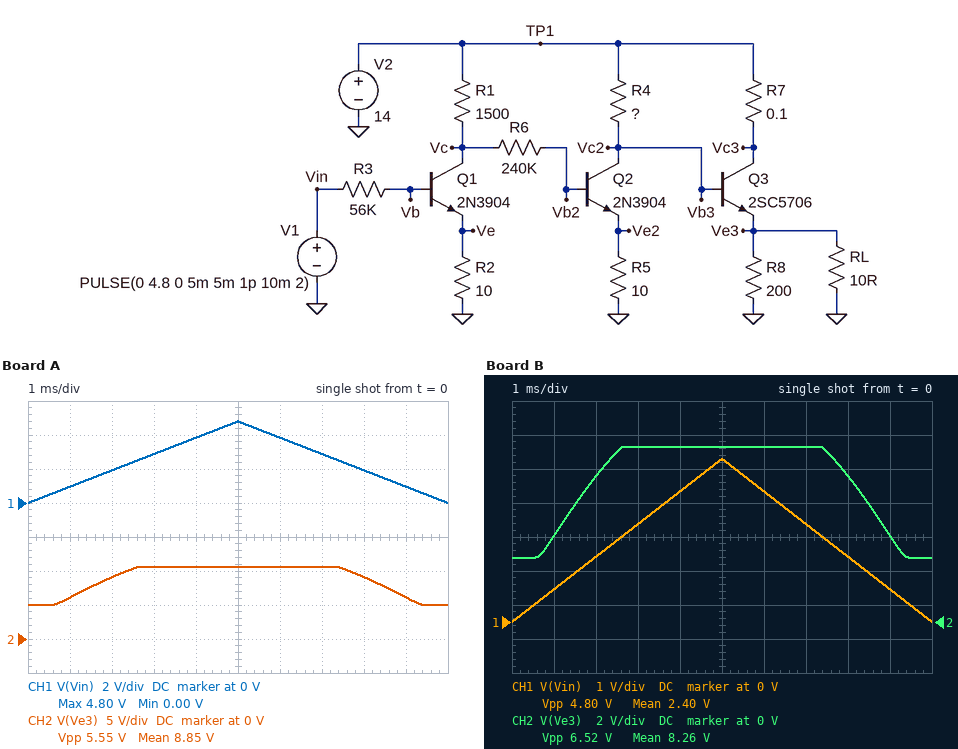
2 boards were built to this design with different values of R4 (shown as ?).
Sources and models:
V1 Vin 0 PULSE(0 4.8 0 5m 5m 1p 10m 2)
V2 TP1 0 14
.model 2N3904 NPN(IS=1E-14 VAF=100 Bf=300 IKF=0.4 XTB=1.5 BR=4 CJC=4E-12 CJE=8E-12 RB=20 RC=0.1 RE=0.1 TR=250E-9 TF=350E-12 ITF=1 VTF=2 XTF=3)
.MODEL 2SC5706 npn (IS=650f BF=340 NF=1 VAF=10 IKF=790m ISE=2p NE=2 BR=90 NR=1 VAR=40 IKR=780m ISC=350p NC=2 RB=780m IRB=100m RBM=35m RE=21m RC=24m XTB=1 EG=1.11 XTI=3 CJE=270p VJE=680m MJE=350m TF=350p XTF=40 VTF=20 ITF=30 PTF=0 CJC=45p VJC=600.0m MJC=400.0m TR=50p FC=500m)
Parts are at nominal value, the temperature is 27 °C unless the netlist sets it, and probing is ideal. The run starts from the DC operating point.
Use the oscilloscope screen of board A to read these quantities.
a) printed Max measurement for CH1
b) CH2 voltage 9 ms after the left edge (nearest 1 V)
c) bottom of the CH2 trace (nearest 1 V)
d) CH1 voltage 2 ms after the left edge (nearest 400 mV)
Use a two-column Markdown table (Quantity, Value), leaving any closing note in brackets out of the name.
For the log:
| Quantity | Value |
|---|---|
| printed Max measurement for CH1 | 4.80 V |
| CH2 voltage 9 ms after the left edge | 6 V |
| bottom of the CH2 trace | 5 V |
| CH1 voltage 2 ms after the left edge | 2.0 V |
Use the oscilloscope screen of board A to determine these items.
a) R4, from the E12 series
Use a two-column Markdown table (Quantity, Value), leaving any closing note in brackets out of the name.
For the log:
| Quantity | Value |
|---|---|
| R4, from the E12 series | 470 Ω |
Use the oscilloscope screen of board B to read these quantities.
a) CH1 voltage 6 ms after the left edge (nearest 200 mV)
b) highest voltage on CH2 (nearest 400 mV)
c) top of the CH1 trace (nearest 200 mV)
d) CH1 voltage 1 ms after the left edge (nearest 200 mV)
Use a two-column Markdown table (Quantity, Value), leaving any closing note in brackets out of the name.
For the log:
| Quantity | Value |
|---|---|
| CH1 voltage 6 ms after the left edge | 3.8 V |
| highest voltage on CH2 | 10.4 V |
| top of the CH1 trace | 4.8 V |
| CH1 voltage 1 ms after the left edge | 1.0 V |
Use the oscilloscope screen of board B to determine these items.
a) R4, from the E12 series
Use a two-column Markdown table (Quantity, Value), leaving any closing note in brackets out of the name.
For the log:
| Quantity | Value |
|---|---|
| R4, from the E12 series | 560 Ω |
